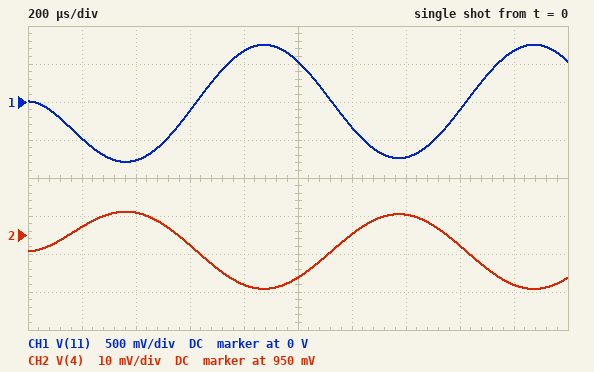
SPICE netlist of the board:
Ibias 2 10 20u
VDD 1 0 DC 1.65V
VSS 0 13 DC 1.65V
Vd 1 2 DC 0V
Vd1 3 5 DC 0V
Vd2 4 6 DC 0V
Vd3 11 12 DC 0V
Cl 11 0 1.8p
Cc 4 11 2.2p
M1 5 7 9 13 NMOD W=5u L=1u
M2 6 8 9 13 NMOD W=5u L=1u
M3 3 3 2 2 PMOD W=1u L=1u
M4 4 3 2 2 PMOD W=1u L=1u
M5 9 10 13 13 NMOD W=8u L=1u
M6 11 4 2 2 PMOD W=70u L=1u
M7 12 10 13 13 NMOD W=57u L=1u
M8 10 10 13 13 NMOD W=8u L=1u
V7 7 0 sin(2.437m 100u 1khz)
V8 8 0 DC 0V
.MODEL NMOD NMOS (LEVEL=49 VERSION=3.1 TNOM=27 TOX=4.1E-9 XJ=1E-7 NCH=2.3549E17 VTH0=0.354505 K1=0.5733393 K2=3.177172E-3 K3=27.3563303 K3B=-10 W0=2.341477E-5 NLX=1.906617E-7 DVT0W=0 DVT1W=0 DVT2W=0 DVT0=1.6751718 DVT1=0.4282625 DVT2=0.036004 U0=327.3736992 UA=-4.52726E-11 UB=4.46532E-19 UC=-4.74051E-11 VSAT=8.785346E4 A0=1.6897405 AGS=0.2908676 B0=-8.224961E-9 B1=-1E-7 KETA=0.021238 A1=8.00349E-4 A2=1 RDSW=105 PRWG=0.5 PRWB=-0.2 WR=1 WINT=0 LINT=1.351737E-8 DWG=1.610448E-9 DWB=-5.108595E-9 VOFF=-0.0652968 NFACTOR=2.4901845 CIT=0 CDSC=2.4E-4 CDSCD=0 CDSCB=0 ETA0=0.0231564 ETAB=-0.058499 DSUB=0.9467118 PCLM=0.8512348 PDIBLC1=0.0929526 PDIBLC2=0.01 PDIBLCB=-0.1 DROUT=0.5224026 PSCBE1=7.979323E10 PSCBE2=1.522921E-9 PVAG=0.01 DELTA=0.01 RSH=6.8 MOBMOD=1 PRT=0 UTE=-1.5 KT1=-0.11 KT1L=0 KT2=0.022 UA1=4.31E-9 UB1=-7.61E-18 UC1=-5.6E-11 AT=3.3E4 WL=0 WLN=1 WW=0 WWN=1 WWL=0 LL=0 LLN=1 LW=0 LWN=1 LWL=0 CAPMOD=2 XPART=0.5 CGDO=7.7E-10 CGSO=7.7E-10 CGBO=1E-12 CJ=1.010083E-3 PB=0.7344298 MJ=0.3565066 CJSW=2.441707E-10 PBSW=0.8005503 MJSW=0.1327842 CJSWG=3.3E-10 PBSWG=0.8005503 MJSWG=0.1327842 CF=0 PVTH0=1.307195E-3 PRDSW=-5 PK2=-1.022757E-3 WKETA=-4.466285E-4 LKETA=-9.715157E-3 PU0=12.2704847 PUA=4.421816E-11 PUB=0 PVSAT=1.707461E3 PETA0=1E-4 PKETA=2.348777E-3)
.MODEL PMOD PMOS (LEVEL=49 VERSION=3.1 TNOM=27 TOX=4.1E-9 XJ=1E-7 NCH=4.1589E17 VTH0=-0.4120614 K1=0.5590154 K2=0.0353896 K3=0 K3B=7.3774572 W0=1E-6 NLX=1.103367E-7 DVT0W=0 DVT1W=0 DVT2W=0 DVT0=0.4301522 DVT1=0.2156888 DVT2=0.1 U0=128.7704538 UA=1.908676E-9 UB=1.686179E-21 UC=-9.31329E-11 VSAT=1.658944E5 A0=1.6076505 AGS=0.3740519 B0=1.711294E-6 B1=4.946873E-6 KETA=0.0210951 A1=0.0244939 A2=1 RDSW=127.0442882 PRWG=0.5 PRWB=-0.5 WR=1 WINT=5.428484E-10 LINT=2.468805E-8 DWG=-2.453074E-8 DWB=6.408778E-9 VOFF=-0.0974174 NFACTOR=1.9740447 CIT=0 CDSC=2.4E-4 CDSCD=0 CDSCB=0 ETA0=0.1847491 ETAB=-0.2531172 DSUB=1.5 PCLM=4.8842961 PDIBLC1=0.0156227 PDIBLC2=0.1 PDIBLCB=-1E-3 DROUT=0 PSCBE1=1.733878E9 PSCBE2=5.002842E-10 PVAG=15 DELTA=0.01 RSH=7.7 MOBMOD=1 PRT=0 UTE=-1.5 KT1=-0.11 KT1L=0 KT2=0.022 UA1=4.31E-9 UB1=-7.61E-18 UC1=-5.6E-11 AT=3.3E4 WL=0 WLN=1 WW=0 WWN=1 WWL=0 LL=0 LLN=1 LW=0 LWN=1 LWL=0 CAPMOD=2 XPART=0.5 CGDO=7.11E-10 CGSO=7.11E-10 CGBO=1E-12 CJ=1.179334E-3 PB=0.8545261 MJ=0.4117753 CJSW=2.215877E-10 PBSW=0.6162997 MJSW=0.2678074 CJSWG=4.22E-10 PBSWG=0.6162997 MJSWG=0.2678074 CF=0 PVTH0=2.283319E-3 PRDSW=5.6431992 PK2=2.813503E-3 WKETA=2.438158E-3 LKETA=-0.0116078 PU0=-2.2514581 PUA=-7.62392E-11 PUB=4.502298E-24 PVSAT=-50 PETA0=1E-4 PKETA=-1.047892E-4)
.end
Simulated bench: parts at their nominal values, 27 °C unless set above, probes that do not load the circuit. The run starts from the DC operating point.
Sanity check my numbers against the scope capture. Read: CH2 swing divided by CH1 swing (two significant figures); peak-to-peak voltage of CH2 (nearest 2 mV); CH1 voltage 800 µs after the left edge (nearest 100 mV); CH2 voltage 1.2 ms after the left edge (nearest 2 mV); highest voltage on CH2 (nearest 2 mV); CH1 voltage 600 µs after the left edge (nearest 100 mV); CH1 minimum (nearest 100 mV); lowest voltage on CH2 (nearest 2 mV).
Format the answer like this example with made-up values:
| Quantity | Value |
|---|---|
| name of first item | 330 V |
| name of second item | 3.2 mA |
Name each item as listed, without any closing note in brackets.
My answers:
| Quantity | Value |
|---|---|
| CH2 swing divided by CH1 swing | 0.013 |
| peak-to-peak voltage of CH2 | 20 mV |
| CH1 voltage 800 µs after the left edge | 700 mV |
| CH2 voltage 1.2 ms after the left edge | 950 mV |
| highest voltage on CH2 | 956 mV |
| CH1 voltage 600 µs after the left edge | -100 mV |
| CH1 minimum | -800 mV |
| lowest voltage on CH2 | 936 mV |
